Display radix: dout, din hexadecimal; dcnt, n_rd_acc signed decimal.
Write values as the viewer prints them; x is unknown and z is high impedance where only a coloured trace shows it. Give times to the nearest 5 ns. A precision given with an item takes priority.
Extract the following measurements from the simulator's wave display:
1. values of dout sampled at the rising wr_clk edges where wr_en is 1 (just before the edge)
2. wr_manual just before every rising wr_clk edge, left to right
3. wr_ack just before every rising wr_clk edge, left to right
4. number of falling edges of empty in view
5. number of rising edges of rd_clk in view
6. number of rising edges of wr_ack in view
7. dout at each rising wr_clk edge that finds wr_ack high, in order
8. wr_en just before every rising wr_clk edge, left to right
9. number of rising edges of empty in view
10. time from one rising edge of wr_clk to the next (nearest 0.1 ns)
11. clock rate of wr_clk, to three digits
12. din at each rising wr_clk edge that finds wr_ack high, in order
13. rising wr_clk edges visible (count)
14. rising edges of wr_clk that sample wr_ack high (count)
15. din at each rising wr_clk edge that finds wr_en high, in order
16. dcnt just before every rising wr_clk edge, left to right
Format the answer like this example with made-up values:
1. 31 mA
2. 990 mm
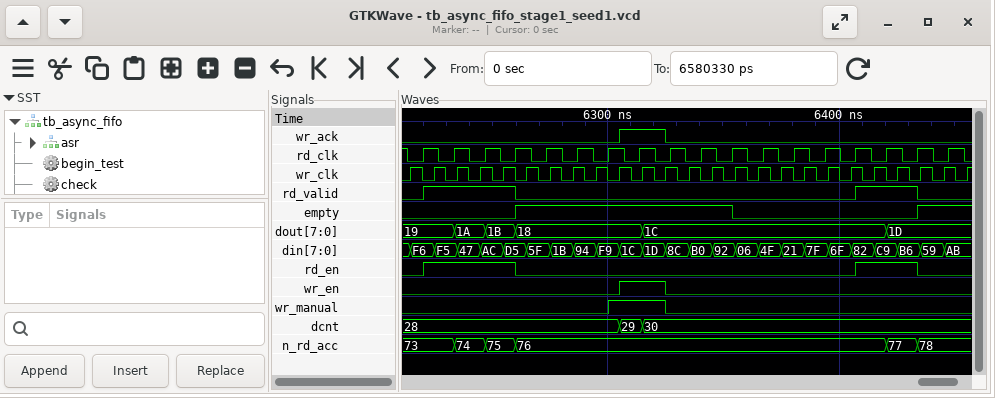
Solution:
1. 18, 1C
2. 0 0 0 0 0 0 0 0 0 1 1 1 0 0 0 0 0 0 0 0 0 0 0 0 0
3. 0 0 0 0 0 0 0 0 0 0 1 1 0 0 0 0 0 0 0 0 0 0 0 0 0
4. 1
5. 18
6. 1
7. 18, 1C
8. 0 0 0 0 0 0 0 0 0 0 1 1 0 0 0 0 0 0 0 0 0 0 0 0 0
9. 2
10. 10 ns
11. 100 MHz
12. 1C, 1D
13. 25
14. 2
15. 1C, 1D
16. 28, 28, 28, 28, 28, 28, 28, 28, 28, 28, 29, 30, 30, 30, 30, 30, 30, 30, 30, 30, 30, 30, 30, 30, 30
